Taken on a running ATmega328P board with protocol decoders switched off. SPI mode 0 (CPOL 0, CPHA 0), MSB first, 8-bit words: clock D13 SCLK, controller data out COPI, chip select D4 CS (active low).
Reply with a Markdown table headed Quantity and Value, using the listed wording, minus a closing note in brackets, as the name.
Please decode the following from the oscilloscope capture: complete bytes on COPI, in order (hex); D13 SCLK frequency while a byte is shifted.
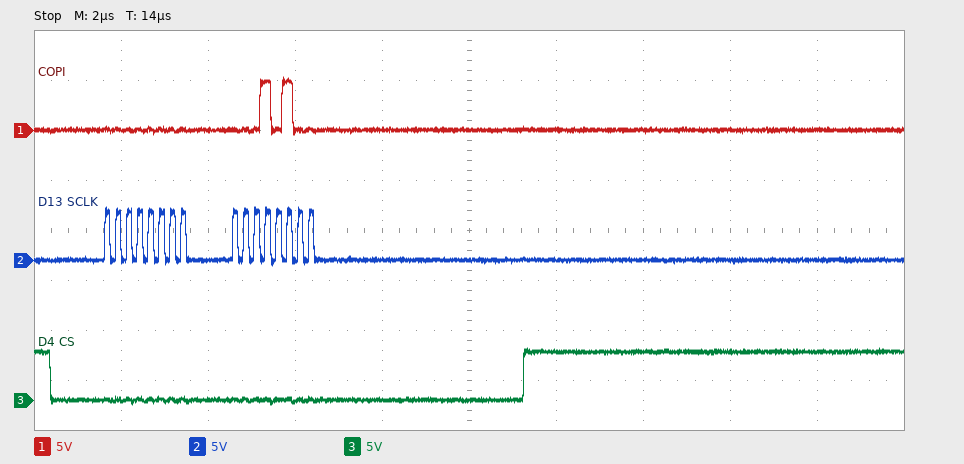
| Quantity | Value |
|---|---|
| complete bytes on COPI, in order | 0x00 0x14 |
| D13 SCLK frequency while a byte is shifted | 4 MHz |
